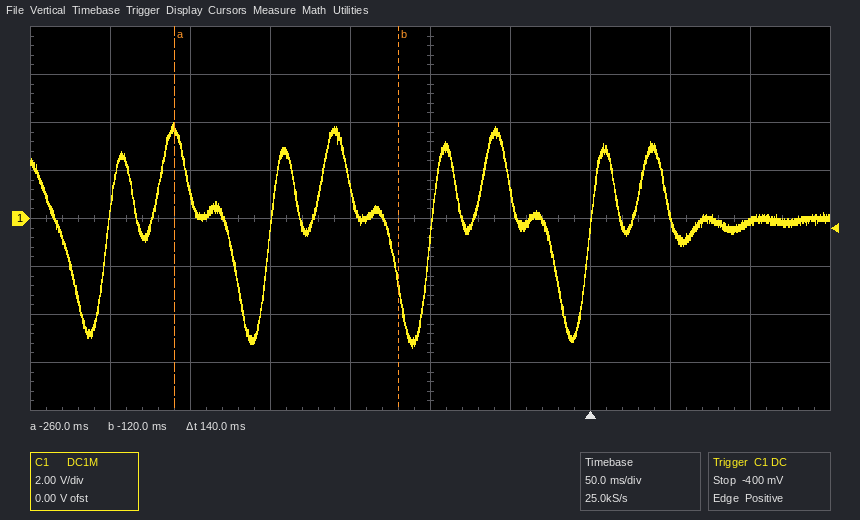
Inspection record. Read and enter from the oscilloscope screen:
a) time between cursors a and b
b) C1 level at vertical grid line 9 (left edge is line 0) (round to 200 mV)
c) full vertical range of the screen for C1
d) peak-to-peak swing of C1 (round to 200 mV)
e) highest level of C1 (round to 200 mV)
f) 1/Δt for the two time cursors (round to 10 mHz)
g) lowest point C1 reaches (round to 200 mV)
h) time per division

140 ms
-200 mV
16 V
9.4 V
4.0 V
7.14 Hz
-5.4 V
50 ms
